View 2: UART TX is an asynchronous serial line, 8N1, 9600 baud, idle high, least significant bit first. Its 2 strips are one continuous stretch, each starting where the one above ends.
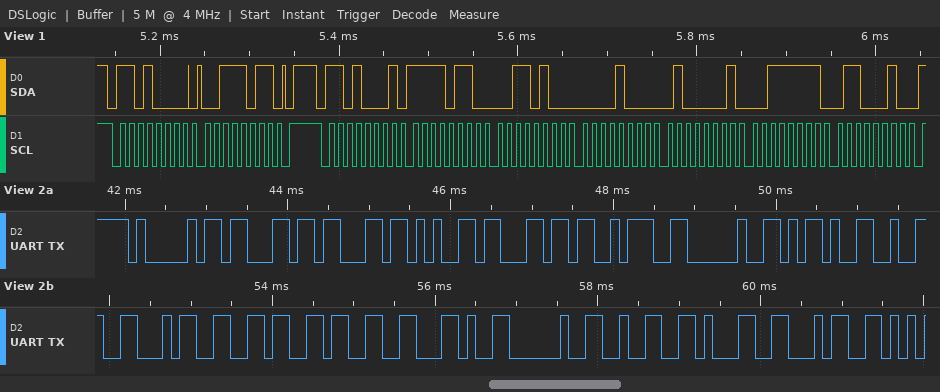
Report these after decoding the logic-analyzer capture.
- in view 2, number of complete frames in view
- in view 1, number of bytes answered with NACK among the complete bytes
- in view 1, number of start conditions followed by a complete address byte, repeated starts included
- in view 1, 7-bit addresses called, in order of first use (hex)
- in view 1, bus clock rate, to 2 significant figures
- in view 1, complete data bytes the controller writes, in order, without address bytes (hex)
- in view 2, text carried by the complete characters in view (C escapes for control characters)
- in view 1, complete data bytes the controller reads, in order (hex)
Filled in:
17
0
2
0x68
100 kHz
3B
"Accel: -2463, 214"
F6 34 08 41 3F 62
